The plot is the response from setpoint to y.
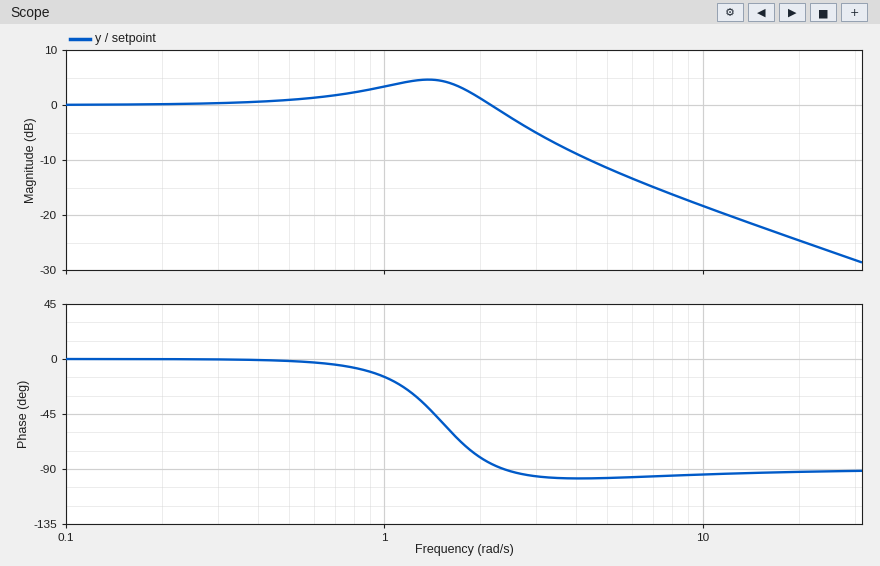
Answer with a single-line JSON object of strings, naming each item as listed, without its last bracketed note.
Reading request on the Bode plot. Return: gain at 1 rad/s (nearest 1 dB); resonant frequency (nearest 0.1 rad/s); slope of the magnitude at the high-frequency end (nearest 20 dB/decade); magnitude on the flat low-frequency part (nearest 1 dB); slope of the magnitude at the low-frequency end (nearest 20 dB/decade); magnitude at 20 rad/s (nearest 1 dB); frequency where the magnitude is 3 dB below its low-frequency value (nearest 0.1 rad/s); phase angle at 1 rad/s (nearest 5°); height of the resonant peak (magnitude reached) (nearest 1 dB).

{"gain at 1 rad/s": "3 dB", "resonant frequency": "1.4 rad/s", "slope of the magnitude at the high-frequency end": "-20 dB/decade", "magnitude on the flat low-frequency part": "0 dB", "slope of the magnitude at the low-frequency end": "0 dB/decade", "magnitude at 20 rad/s": "-25 dB", "frequency where the magnitude is 3 dB below its low-frequency value": "2.6 rad/s", "phase angle at 1 rad/s": "-15°", "height of the resonant peak (magnitude reached)": "5 dB"}
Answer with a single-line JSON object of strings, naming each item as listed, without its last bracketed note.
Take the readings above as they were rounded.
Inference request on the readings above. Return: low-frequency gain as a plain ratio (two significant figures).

{"low-frequency gain as a plain ratio": "1.0"}
